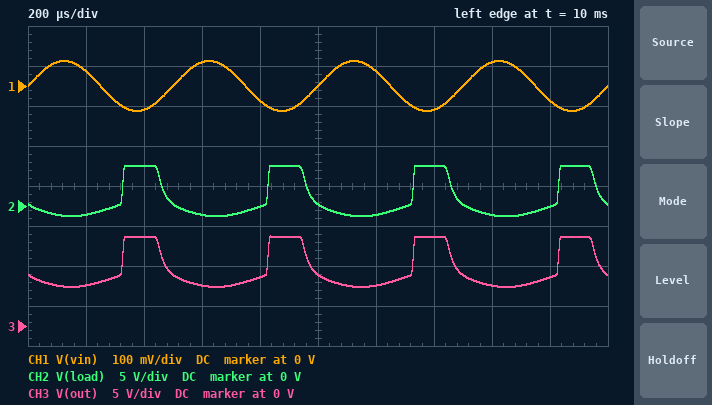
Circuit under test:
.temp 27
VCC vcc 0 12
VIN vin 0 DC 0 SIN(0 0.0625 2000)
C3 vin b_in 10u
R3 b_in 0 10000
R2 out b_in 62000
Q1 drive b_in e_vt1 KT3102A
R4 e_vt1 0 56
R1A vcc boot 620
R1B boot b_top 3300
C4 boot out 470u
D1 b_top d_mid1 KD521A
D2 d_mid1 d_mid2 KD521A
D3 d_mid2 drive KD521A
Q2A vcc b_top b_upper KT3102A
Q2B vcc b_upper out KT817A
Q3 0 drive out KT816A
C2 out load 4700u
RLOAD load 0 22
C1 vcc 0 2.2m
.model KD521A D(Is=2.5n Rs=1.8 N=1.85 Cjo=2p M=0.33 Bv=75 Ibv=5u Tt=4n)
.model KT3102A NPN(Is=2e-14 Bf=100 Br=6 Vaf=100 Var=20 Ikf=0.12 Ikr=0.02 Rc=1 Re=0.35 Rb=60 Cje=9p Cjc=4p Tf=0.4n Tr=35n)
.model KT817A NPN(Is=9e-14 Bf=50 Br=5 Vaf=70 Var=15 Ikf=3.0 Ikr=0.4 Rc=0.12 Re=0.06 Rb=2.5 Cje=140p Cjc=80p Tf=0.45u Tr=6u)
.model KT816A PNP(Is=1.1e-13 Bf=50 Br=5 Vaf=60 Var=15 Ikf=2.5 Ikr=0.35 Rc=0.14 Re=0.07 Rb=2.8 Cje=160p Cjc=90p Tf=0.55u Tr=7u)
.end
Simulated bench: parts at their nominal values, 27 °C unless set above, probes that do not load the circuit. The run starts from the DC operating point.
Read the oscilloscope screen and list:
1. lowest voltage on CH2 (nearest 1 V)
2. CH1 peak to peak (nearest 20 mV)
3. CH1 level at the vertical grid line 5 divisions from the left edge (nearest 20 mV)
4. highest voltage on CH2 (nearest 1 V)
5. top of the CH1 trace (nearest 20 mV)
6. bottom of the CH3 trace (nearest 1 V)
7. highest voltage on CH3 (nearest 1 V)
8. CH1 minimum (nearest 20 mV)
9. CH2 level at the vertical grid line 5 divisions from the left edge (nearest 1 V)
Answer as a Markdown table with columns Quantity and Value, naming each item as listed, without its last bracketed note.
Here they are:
| Quantity | Value |
|---|---|
| lowest voltage on CH2 | -1 V |
| CH1 peak to peak | 120 mV |
| CH1 level at the vertical grid line 5 divisions from the left edge | 0 V |
| highest voltage on CH2 | 5 V |
| top of the CH1 trace | 60 mV |
| bottom of the CH3 trace | 5 V |
| highest voltage on CH3 | 11 V |
| CH1 minimum | -60 mV |
| CH2 level at the vertical grid line 5 divisions from the left edge | 0 V |
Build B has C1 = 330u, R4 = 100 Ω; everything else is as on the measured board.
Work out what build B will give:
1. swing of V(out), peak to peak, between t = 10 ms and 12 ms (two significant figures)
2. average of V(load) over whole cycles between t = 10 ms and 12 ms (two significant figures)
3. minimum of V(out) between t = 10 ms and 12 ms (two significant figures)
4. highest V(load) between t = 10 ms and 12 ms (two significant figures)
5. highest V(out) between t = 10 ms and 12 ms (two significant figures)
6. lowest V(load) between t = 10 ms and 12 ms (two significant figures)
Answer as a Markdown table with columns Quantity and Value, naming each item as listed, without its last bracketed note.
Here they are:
| Quantity | Value |
|---|---|
| swing of V(out), peak to peak, between t = 10 ms and 12 ms | 5.5 V |
| average of V(load) over whole cycles between t = 10 ms and 12 ms | 780 mV |
| minimum of V(out) between t = 10 ms and 12 ms | 5.6 V |
| highest V(load) between t = 10 ms and 12 ms | 4.7 V |
| highest V(out) between t = 10 ms and 12 ms | 11 V |
| lowest V(load) between t = 10 ms and 12 ms | -810 mV |
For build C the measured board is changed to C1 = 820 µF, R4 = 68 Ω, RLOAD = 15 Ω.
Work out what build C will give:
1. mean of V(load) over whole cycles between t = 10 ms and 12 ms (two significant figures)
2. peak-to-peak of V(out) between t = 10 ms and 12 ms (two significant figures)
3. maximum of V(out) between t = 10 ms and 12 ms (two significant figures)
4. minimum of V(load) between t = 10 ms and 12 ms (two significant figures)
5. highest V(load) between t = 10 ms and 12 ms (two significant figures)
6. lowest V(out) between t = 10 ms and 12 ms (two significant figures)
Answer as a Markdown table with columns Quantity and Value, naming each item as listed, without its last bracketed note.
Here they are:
| Quantity | Value |
|---|---|
| mean of V(load) over whole cycles between t = 10 ms and 12 ms | 860 mV |
| peak-to-peak of V(out) between t = 10 ms and 12 ms | 5.6 V |
| maximum of V(out) between t = 10 ms and 12 ms | 11 V |
| minimum of V(load) between t = 10 ms and 12 ms | -790 mV |
| highest V(load) between t = 10 ms and 12 ms | 4.8 V |
| lowest V(out) between t = 10 ms and 12 ms | 5.5 V |
